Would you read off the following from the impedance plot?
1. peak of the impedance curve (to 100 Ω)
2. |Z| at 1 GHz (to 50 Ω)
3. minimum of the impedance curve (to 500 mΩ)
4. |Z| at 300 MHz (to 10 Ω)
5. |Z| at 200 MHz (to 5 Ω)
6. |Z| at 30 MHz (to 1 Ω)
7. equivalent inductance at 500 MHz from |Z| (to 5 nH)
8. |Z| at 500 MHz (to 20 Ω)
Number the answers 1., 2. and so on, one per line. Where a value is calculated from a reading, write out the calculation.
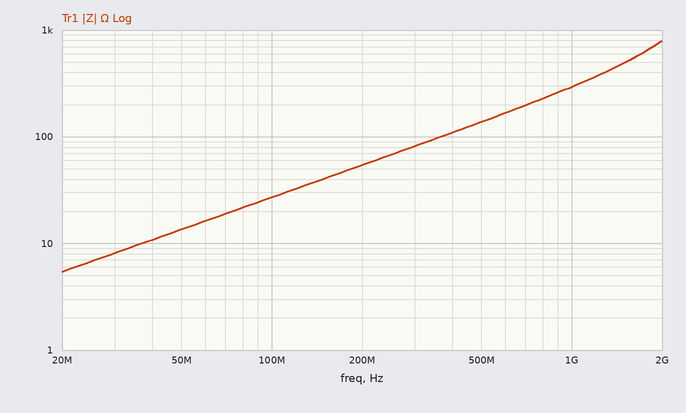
1. 800 Ω
2. 300 Ω
3. 5.5 Ω
4. 80 Ω
5. 55 Ω
6. 8 Ω
7. L = 140 Ω/(2π × 500 MHz) ≈ 45 nH
8. 140 Ω
